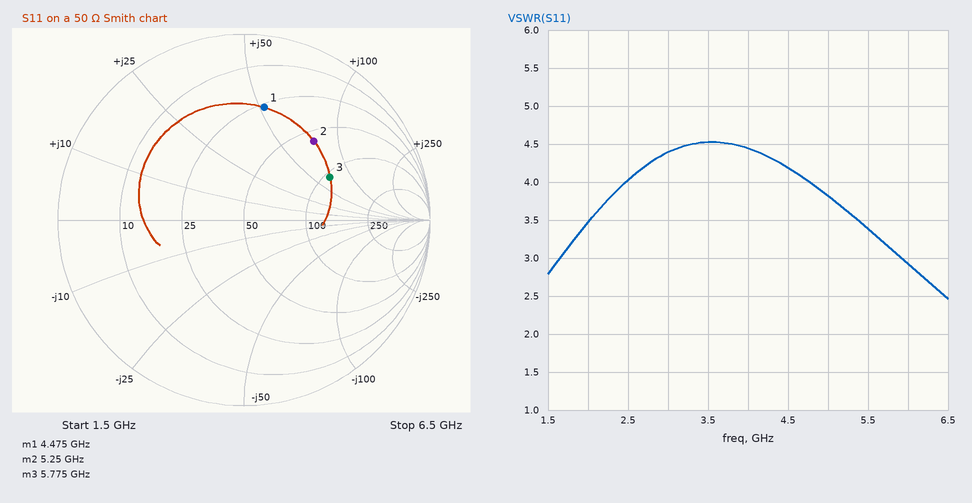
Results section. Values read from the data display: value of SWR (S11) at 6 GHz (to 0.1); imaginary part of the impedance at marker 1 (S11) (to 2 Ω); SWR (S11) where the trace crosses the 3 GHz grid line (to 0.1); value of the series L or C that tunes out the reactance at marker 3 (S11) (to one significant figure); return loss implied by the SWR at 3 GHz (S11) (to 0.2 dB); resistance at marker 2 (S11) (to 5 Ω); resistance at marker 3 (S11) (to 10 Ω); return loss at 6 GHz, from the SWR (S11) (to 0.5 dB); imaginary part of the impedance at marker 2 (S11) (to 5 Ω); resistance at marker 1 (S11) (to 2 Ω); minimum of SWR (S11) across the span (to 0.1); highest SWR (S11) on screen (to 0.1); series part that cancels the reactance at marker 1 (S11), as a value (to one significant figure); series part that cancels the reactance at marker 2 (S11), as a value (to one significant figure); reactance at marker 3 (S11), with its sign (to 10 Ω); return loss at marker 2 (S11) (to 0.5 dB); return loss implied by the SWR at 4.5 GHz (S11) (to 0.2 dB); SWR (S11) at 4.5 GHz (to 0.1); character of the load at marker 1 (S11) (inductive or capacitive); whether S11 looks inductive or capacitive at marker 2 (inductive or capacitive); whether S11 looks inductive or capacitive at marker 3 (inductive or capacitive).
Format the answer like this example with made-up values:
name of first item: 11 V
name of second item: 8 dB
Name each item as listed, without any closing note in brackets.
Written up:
value of SWR (S11) at 6 GHz: 2.9
imaginary part of the impedance at marker 1 (S11): +52 Ω
SWR (S11) where the trace crosses the 3 GHz grid line: 4.4
value of the series L or C that tunes out the reactance at marker 3 (S11): 400 fF
return loss implied by the SWR at 3 GHz (S11): 4.0 dB
resistance at marker 2 (S11): 60 Ω
resistance at marker 3 (S11): 110 Ω
return loss at 6 GHz, from the SWR (S11): 6.0 dB
imaginary part of the impedance at marker 2 (S11): +75 Ω
resistance at marker 1 (S11): 26 Ω
minimum of SWR (S11) across the span: 2.5
highest SWR (S11) on screen: 4.5
series part that cancels the reactance at marker 1 (S11), as a value: 700 fF
series part that cancels the reactance at marker 2 (S11), as a value: 400 fF
reactance at marker 3 (S11), with its sign: +70 Ω
return loss at marker 2 (S11): 5.0 dB
return loss implied by the SWR at 4.5 GHz (S11): 4.2 dB
SWR (S11) at 4.5 GHz: 4.2
character of the load at marker 1 (S11): inductive
whether S11 looks inductive or capacitive at marker 2: inductive
whether S11 looks inductive or capacitive at marker 3: inductive
